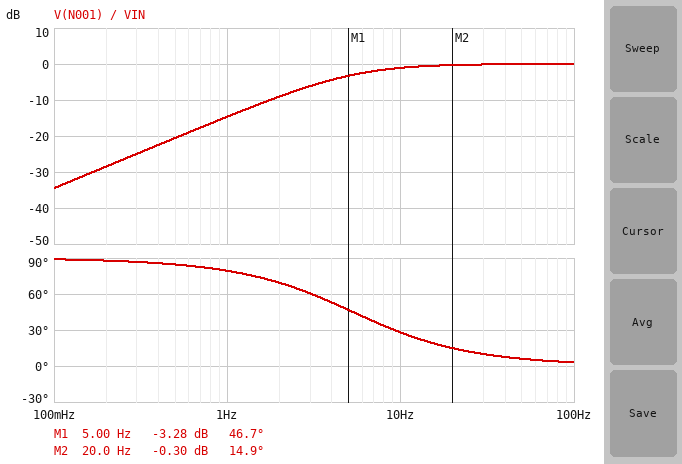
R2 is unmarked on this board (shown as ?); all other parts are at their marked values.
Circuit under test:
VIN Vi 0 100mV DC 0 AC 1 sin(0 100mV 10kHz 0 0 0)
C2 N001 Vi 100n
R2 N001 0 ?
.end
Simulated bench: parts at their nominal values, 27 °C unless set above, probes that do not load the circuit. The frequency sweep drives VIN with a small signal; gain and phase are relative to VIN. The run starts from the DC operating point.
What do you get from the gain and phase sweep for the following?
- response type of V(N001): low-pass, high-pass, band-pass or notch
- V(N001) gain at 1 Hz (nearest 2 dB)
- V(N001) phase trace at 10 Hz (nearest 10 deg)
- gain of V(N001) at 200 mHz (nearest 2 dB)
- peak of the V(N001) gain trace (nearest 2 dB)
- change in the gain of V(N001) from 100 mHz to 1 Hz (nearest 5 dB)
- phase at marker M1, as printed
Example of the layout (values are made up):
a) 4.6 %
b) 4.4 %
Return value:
a) high-pass
b) -14 dB
c) 30 deg
d) -28 dB
e) 0 dB
f) 20 dB
g) 46.7 deg
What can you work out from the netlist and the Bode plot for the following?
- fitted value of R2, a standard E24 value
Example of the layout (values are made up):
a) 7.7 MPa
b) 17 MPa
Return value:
a) 300 kΩ
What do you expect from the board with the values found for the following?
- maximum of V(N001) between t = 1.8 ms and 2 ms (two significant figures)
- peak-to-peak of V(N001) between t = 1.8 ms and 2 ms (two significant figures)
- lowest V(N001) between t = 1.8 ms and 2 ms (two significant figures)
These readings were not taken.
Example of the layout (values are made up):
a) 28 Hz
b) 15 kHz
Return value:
a) 100 mV
b) 200 mV
c) -100 mV
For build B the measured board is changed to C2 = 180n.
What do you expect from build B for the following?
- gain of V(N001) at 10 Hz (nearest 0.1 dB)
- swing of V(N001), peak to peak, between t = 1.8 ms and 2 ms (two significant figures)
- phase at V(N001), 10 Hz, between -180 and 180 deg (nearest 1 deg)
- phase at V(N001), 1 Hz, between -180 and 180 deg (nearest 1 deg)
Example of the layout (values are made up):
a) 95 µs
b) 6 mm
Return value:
a) -0.4 dB
b) 200 mV
c) 16 deg
d) 71 deg
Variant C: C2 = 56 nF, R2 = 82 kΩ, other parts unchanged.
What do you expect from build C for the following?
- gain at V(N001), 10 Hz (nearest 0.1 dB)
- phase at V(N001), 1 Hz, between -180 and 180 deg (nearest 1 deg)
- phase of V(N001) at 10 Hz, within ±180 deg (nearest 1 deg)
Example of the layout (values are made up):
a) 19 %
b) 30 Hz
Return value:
a) -11.1 dB
b) 88 deg
c) 74 deg
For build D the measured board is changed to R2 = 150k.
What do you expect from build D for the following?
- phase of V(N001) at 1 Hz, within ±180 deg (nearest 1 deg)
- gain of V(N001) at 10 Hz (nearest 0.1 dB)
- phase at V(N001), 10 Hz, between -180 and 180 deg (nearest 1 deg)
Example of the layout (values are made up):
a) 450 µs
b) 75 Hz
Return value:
a) 85 deg
b) -3.3 dB
c) 47 deg
